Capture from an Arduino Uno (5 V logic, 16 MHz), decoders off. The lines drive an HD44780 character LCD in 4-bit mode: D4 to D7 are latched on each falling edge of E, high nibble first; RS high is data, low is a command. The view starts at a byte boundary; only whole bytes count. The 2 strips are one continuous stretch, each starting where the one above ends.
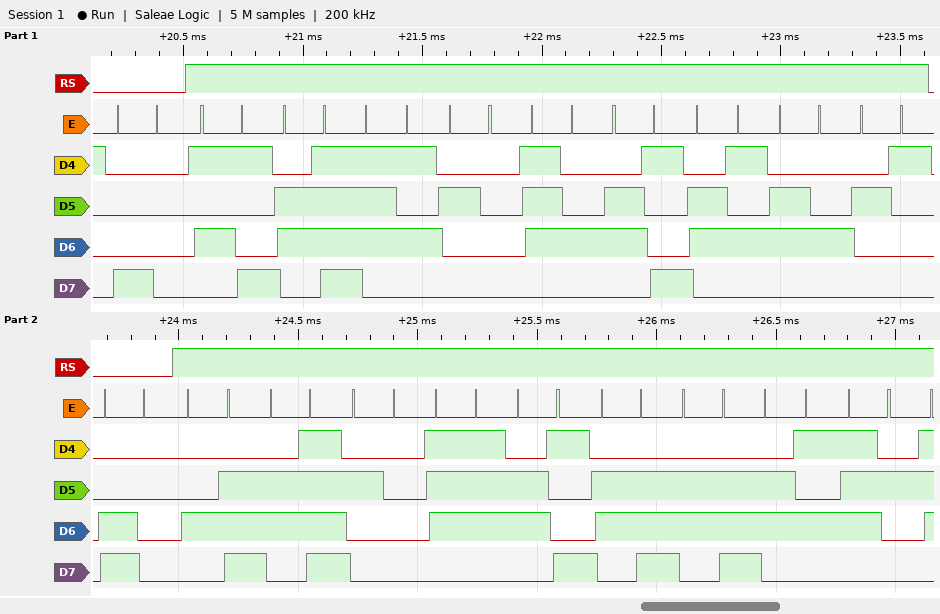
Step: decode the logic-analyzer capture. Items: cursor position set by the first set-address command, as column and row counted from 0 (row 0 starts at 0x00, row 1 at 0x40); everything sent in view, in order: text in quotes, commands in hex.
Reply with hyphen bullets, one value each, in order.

- column 0, row 0
- 0x80 "You tied!" 0xC0 "No winner"
